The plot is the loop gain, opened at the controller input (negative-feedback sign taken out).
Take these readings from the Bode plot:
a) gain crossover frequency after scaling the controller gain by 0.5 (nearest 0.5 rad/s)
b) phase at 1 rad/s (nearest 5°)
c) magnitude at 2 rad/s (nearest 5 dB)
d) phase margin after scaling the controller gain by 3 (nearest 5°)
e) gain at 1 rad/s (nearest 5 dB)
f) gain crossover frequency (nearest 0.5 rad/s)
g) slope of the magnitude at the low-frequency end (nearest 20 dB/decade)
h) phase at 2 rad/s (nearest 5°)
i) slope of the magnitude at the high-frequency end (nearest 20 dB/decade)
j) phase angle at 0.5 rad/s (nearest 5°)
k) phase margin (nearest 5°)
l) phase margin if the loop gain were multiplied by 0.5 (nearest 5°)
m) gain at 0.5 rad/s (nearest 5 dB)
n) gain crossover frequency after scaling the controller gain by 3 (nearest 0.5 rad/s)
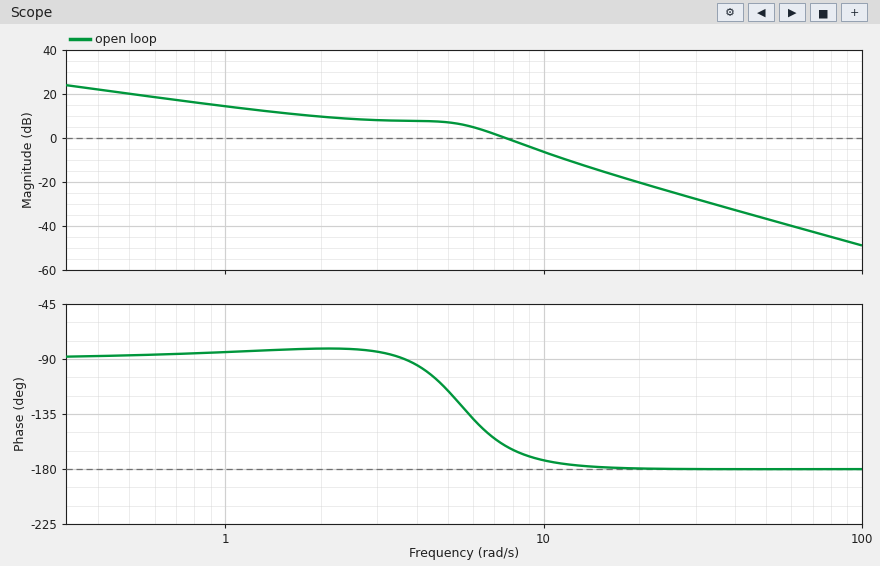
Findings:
5.5 rad/s
-85°
10 dB
5°
15 dB
7.5 rad/s
-20 dB/decade
-80°
-40 dB/decade
-85°
20°
50°
20 dB
11.5 rad/s
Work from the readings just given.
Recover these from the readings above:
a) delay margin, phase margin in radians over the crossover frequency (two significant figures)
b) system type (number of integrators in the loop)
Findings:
0.047 s
1
